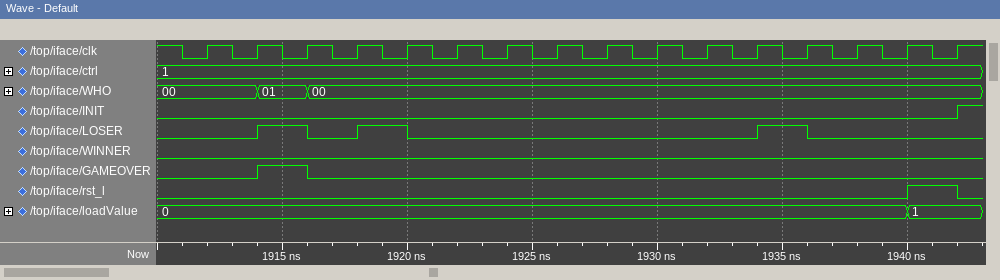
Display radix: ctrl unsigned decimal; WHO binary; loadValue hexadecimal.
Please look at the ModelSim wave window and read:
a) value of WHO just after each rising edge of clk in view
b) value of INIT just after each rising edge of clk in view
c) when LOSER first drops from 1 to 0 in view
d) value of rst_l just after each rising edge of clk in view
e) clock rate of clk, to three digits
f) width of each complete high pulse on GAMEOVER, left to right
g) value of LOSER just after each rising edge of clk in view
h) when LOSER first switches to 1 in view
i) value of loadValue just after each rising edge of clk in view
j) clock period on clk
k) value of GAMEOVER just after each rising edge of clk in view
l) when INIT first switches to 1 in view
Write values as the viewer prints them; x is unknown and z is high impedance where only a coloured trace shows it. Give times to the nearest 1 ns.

00, 01, 00, 00, 00, 00, 00, 00, 00, 00, 00, 00, 00, 00, 00, 00
0 0 0 0 0 0 0 0 0 0 0 0 0 0 0 1
1916 ns
0 0 0 0 0 0 0 0 0 0 0 0 0 0 1 0
500 MHz
2 ns
0 1 0 1 0 0 0 0 0 0 0 1 0 0 0 0
1914 ns
0, 0, 0, 0, 0, 0, 0, 0, 0, 0, 0, 0, 0, 0, 1, 1
2 ns
0 1 0 0 0 0 0 0 0 0 0 0 0 0 0 0
1942 ns
